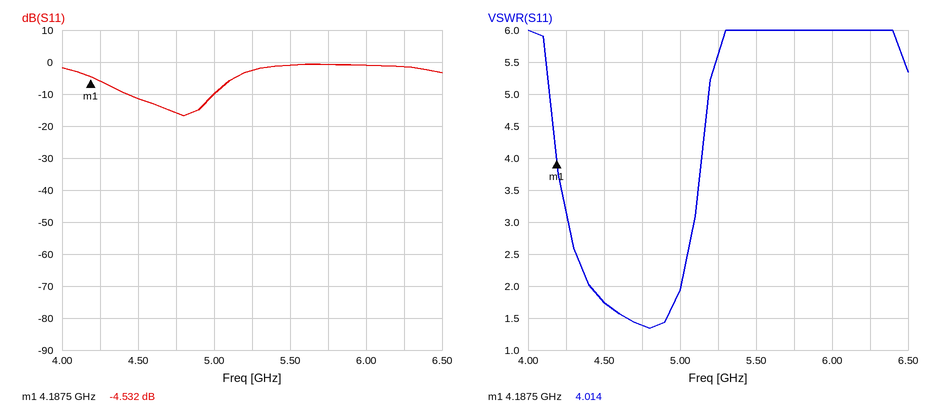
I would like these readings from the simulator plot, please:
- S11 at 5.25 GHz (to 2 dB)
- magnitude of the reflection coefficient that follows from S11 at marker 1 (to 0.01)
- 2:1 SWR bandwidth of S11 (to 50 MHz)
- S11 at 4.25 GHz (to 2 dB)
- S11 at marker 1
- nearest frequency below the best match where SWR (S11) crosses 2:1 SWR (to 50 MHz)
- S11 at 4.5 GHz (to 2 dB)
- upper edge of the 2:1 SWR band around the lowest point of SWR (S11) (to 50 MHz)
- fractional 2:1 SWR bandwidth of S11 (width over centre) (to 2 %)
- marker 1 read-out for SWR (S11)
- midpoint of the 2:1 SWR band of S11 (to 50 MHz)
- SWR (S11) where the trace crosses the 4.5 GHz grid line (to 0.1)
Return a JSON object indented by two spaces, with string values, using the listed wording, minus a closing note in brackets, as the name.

{
  "S11 at 5.25 GHz": "-2 dB",
  "magnitude of the reflection coefficient that follows from S11 at marker 1": "0.59",
  "2:1 SWR bandwidth of S11": "600 MHz",
  "S11 at 4.25 GHz": "-6 dB",
  "S11 at marker 1": "-4.532 dB",
  "nearest frequency below the best match where SWR (S11) crosses 2:1 SWR": "4.40 GHz",
  "S11 at 4.5 GHz": "-12 dB",
  "upper edge of the 2:1 SWR band around the lowest point of SWR (S11)": "5.00 GHz",
  "fractional 2:1 SWR bandwidth of S11 (width over centre)": "12 %",
  "marker 1 read-out for SWR": "4.014",
  "midpoint of the 2:1 SWR band of S11": "4.70 GHz",
  "SWR (S11) where the trace crosses the 4.5 GHz grid line": "1.7"
}
